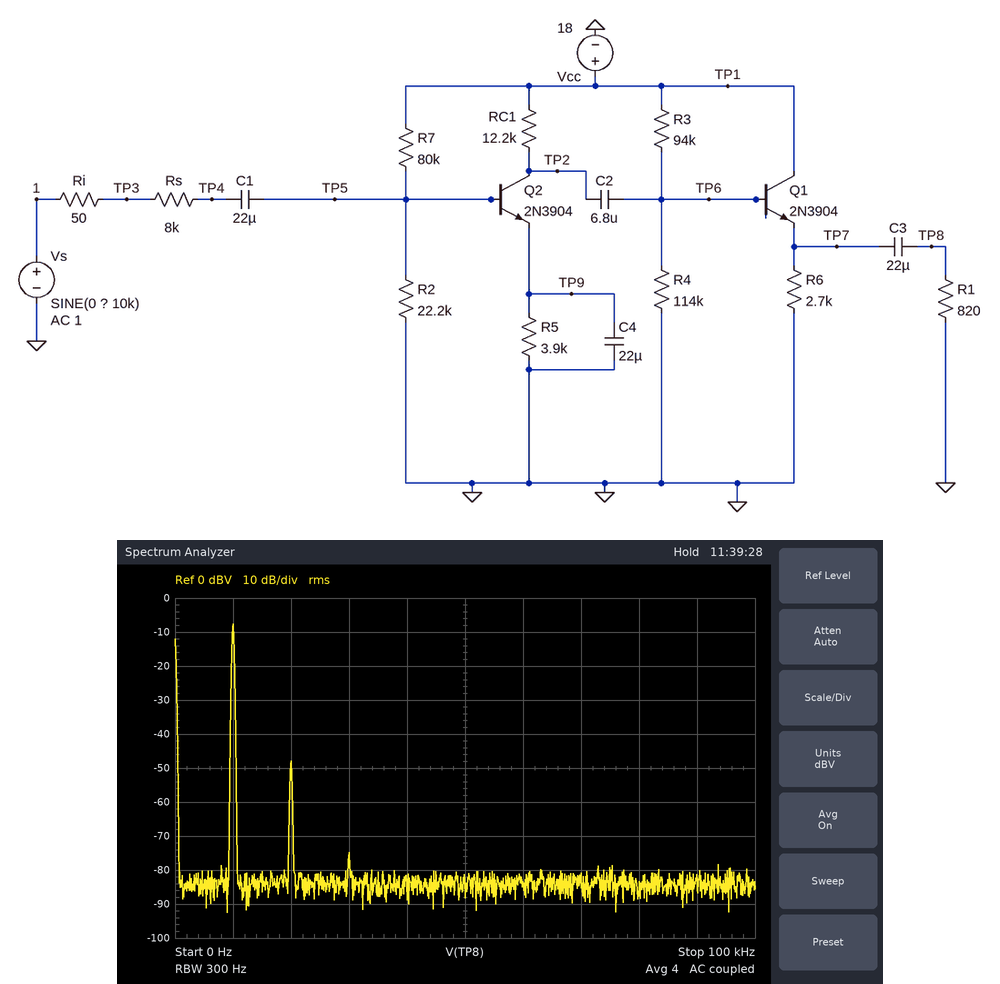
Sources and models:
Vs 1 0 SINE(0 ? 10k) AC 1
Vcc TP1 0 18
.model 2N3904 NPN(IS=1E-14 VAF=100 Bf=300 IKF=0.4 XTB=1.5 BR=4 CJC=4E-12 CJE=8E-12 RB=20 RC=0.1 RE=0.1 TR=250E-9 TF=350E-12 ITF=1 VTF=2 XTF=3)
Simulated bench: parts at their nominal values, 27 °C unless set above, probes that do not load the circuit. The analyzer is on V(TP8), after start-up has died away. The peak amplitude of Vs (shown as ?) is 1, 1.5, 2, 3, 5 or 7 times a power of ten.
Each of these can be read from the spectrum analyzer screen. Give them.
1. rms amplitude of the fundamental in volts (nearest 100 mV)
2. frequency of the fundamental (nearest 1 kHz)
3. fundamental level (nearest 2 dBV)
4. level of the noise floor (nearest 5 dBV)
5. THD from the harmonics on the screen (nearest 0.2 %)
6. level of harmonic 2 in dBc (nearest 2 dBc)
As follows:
400 mV
10 kHz
-8 dBV
-85 dBV
1.0 %
-40 dBc
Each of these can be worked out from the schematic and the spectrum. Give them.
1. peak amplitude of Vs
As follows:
5 mV
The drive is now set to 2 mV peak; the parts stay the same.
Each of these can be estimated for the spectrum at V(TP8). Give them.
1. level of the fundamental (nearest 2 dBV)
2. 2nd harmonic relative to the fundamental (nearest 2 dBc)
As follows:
-16 dBV
-48 dBc
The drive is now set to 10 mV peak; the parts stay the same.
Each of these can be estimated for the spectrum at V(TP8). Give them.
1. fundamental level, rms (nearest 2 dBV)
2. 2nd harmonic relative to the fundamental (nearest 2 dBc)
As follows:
-2 dBV
-34 dBc
